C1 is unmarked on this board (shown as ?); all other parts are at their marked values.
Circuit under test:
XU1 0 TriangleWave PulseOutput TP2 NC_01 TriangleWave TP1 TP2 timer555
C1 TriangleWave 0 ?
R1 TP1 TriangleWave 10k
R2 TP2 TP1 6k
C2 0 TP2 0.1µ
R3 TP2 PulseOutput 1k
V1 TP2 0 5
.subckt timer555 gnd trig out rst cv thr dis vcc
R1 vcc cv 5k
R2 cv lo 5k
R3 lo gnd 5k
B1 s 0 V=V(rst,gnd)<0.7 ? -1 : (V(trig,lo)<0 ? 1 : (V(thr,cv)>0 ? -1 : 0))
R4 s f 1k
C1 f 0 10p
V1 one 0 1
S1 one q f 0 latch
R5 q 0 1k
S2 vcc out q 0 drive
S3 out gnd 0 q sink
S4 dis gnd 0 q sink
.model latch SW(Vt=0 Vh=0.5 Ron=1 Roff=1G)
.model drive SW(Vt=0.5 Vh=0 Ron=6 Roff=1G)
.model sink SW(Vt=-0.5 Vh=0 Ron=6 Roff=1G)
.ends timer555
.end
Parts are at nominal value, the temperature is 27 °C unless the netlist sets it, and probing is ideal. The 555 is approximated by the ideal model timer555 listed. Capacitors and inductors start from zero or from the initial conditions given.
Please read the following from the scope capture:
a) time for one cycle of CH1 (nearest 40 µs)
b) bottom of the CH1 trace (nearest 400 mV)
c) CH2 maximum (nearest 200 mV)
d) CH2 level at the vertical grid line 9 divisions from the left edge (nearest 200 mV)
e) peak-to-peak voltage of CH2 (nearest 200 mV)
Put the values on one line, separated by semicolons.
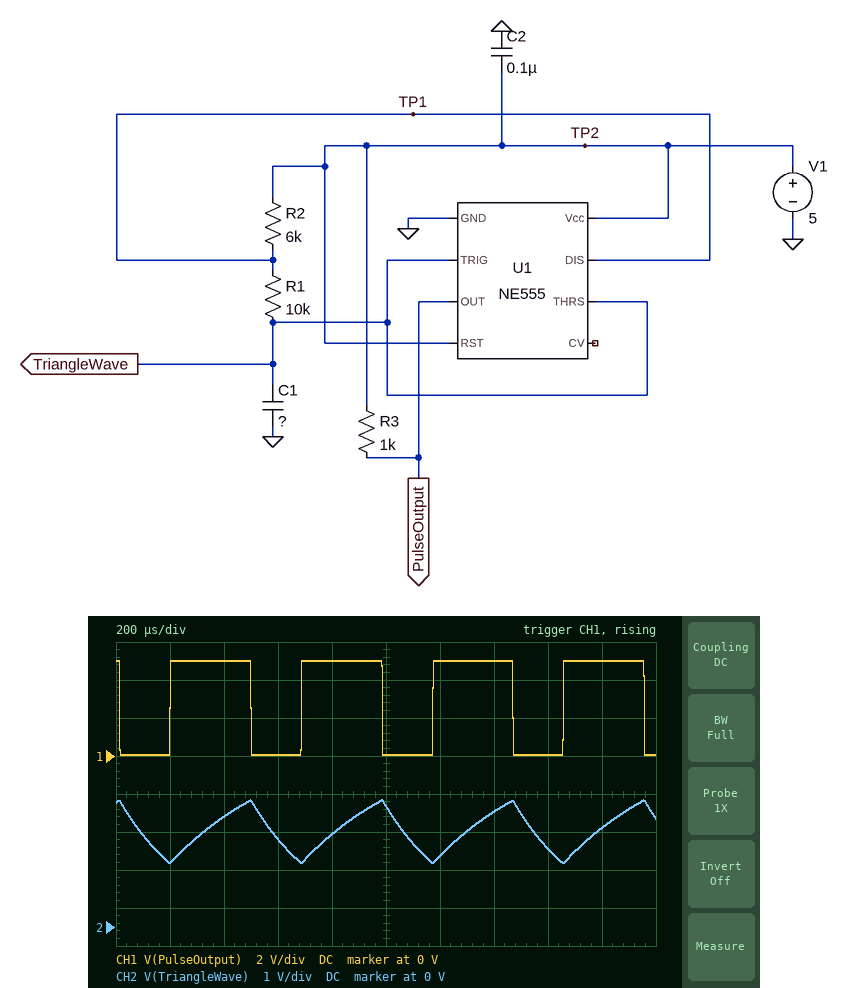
480 µs; 0 V; 3.4 V; 2.6 V; 1.6 V
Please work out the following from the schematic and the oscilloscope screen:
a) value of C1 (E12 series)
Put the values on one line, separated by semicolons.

27 nF
